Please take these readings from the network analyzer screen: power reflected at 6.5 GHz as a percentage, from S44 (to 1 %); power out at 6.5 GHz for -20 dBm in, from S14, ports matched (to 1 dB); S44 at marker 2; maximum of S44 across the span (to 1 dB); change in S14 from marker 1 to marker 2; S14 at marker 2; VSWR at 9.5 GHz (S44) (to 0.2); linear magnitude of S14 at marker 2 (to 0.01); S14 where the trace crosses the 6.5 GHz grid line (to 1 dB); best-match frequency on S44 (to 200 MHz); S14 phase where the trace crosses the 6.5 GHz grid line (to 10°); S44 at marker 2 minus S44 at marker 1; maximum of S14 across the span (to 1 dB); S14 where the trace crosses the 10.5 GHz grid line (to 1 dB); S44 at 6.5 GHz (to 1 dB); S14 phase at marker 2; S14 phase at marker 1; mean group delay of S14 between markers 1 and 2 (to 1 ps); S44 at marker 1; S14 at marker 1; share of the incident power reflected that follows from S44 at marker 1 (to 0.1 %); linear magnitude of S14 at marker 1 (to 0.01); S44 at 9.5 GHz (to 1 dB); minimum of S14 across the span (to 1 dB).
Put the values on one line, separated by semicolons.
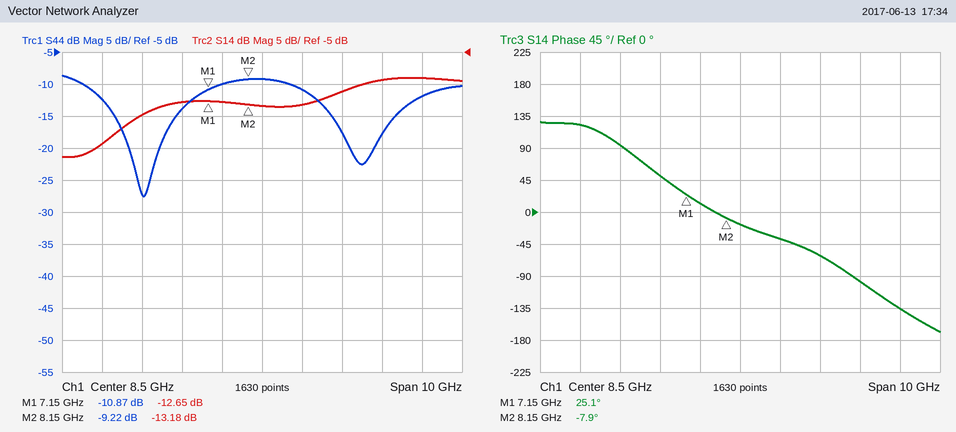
4 %; -33 dBm; -9.22 dB; -9 dB; -0.53 dB; -13.18 dB; 1.8; 0.22; -13 dB; 5.6 GHz; 50°; 1.65 dB; -9 dB; -11 dB; -14 dB; -7.9°; 25.1°; 92 ps; -10.87 dB; -12.65 dB; 8.2 %; 0.23; -11 dB; -21 dB
